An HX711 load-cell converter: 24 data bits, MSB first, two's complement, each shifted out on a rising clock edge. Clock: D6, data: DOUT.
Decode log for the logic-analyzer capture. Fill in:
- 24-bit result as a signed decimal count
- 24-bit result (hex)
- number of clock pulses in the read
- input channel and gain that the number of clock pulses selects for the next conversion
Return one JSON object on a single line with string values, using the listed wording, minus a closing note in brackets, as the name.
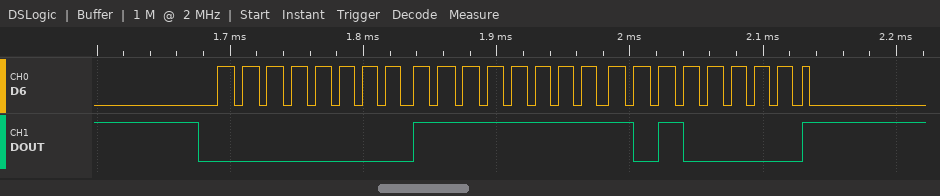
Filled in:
{"24-bit result as a signed decimal count": "65440", "24-bit result": "0x00FFA0", "number of clock pulses in the read": "25", "input channel and gain that the number of clock pulses selects for the next conversion": "channel A, gain 128"}
